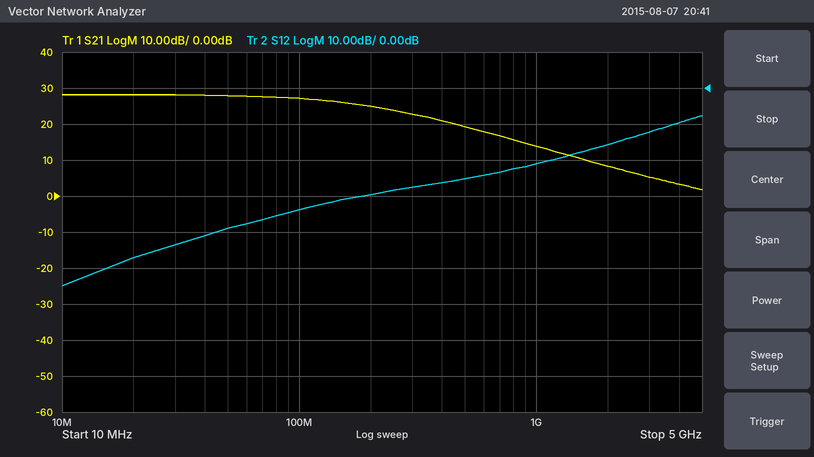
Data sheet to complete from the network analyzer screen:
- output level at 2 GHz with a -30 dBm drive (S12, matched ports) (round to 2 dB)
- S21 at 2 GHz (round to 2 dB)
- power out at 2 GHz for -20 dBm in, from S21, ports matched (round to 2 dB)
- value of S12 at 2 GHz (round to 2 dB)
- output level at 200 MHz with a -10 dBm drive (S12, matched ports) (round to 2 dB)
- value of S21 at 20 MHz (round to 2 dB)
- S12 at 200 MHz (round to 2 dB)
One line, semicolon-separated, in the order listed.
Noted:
-46 dBm; 8 dB; -12 dBm; -16 dB; -40 dBm; 28 dB; -30 dB
